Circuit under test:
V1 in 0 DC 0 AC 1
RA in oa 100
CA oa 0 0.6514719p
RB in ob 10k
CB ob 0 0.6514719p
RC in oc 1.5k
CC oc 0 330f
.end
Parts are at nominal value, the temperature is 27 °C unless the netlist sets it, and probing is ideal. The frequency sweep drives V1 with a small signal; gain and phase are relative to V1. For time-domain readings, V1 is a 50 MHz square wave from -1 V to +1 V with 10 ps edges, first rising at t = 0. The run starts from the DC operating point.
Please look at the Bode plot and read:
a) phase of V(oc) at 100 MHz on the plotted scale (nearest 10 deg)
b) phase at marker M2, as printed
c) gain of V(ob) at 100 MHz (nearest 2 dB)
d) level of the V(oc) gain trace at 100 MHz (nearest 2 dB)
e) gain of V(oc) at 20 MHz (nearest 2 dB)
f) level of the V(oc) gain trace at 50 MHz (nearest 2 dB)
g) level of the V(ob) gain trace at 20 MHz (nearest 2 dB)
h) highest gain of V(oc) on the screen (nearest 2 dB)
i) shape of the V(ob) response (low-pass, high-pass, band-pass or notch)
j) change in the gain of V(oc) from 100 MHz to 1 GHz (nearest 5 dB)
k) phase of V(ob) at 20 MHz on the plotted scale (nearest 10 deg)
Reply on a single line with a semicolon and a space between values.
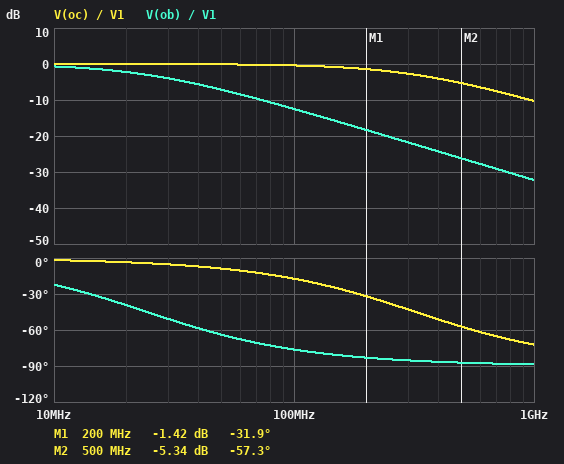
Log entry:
-20 deg; -57.3 deg; -12 dB; 0 dB; 0 dB; 0 dB; -2 dB; 0 dB; low-pass; -10 dB; -40 deg
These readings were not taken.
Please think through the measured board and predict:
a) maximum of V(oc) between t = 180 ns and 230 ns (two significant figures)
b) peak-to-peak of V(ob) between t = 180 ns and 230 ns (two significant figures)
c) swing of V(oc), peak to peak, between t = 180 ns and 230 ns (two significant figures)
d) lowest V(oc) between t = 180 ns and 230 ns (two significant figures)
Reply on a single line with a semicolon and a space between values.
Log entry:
1.0 V; 1.3 V; 2.0 V; -1.0 V
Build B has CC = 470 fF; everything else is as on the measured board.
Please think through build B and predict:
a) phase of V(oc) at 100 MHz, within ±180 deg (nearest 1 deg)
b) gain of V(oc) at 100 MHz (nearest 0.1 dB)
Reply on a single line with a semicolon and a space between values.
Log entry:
-24 deg; -0.8 dB
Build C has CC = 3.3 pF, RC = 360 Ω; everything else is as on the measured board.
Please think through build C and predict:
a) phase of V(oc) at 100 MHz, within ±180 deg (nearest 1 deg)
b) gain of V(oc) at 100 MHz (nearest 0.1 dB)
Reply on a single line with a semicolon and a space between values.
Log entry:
-37 deg; -1.9 dB
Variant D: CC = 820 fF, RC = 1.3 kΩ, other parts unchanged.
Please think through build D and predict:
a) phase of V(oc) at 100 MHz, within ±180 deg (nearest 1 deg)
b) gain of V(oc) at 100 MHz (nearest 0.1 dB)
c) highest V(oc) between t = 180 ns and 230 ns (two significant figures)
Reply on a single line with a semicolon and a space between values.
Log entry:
-34 deg; -1.6 dB; 1.0 V
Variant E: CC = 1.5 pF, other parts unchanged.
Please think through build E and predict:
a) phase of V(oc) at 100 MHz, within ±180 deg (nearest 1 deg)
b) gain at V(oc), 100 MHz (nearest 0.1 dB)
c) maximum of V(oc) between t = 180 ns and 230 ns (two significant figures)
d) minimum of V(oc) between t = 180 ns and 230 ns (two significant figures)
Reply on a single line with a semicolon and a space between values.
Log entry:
-55 deg; -4.8 dB; 980 mV; -980 mV
